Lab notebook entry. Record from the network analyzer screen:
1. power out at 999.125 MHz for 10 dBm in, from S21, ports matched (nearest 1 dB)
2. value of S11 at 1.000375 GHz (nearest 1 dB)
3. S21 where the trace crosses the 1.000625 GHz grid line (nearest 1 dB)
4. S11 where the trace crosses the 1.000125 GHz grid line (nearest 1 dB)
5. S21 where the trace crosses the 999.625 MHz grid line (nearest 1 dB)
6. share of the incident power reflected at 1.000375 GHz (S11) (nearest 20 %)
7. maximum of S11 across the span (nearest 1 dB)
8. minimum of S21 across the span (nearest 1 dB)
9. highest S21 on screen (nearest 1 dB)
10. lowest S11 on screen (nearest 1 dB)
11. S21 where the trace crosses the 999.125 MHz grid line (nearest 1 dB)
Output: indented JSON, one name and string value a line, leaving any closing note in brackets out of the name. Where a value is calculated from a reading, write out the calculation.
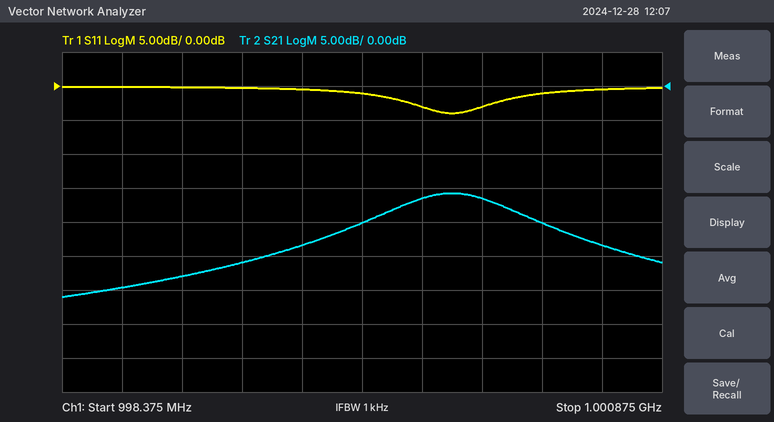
{
  "power out at 999.125 MHz for 10 dBm in, from S21, ports matched": "10 dBm + (-26 dB) = -16 dBm",
  "value of S11 at 1.000375 GHz": "-1 dB",
  "S21 where the trace crosses the 1.000625 GHz grid line": "-23 dB",
  "S11 where the trace crosses the 1.000125 GHz grid line": "-3 dB",
  "S21 where the trace crosses the 999.625 MHz grid line": "-20 dB",
  "share of the incident power reflected at 1.000375 GHz (S11)": "10^(-1/10) ≈ 79.4 %, so 80 % to the nearest 20 %",
  "maximum of S11 across the span": "0 dB",
  "minimum of S21 across the span": "-31 dB",
  "highest S21 on screen": "-16 dB",
  "lowest S11 on screen": "-4 dB",
  "S21 where the trace crosses the 999.125 MHz grid line": "-26 dB"
}
